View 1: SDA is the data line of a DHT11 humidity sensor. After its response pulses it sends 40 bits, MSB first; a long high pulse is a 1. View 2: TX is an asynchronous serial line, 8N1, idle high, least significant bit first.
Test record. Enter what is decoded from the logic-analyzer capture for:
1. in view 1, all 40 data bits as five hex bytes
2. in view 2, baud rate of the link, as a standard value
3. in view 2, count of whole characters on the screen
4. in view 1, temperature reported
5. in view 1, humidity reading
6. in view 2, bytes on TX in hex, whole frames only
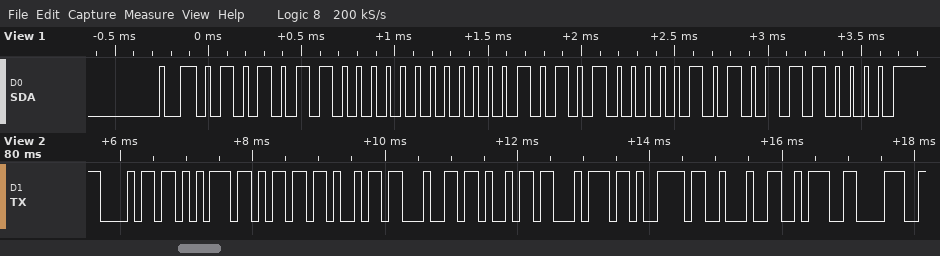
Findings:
56 00 15 05 70
9600 baud
11
21.5 °C
86 %
68 75 6D 69 64 69 74 79 22 3A 38
